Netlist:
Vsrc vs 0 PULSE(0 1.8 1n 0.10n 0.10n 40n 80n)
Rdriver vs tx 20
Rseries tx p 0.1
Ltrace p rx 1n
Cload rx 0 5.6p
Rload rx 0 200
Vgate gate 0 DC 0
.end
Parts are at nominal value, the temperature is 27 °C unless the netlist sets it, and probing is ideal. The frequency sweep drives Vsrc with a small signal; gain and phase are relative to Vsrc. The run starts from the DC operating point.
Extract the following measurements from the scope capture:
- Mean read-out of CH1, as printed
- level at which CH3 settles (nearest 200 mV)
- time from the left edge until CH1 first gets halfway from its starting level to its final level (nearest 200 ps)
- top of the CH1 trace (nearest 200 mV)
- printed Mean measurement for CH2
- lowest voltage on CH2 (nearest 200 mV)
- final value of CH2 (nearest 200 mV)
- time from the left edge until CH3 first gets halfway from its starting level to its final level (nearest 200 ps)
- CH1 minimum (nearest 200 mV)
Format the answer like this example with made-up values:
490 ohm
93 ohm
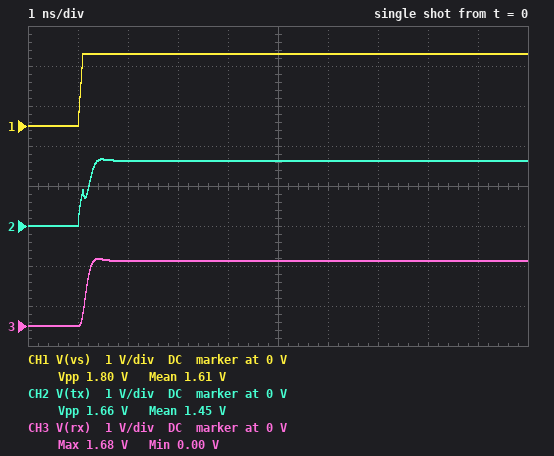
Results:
1.61 V
1.6 V
1.0 ns
1.8 V
1.45 V
0 V
1.6 V
1.2 ns
0 V
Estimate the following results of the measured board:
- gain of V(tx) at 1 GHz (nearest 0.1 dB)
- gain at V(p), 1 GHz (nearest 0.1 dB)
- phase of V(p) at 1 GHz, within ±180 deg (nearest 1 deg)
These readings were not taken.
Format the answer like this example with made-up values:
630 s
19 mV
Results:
-3.4 dB
-3.4 dB
-38 deg
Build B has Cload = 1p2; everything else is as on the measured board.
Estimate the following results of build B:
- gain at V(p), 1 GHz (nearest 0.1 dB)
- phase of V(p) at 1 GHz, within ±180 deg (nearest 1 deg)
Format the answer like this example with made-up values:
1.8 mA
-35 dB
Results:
-1.0 dB
-8 deg
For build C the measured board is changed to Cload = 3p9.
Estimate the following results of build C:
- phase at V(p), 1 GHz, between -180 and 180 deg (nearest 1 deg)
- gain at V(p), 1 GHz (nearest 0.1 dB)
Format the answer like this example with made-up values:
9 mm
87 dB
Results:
-27 deg
-2.1 dB
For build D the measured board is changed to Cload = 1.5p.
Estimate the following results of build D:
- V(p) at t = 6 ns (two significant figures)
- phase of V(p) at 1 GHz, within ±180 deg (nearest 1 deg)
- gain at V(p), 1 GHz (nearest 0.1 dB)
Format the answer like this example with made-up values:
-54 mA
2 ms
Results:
1.6 V
-10 deg
-1.1 dB
